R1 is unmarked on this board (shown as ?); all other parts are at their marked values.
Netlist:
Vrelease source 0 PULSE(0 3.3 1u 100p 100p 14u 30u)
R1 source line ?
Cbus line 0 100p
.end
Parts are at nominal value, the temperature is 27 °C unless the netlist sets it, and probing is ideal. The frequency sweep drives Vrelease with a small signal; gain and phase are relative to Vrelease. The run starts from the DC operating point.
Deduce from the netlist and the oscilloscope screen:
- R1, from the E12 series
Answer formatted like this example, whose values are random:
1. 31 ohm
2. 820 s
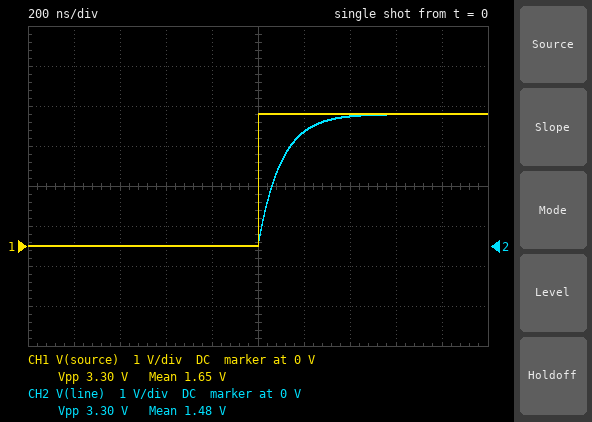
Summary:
1. 1 kΩ
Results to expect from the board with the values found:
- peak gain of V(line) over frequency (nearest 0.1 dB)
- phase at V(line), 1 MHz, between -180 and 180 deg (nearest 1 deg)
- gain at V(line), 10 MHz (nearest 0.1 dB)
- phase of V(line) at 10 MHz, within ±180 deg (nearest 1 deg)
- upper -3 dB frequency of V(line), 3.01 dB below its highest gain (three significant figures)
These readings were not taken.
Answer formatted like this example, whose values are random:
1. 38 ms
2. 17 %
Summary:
1. 0 dB
2. -32 deg
3. -16.1 dB
4. -81 deg
5. 1.59 MHz
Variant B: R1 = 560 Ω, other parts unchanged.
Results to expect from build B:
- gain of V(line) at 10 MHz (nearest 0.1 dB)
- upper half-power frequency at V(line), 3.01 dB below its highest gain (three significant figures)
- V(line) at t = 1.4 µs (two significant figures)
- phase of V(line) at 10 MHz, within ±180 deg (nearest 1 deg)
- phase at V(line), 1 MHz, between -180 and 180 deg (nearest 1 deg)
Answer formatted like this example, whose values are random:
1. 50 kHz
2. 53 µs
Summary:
1. -11.3 dB
2. 2.84 MHz
3. 3.3 V
4. -74 deg
5. -19 deg
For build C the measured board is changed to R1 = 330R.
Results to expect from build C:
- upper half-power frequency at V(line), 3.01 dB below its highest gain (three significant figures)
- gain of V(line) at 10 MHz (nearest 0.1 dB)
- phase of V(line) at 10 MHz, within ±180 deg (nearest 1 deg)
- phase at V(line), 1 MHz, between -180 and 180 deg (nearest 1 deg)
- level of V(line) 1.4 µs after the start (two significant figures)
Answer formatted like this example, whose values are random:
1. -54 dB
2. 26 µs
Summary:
1. 4.82 MHz
2. -7.2 dB
3. -64 deg
4. -12 deg
5. 3.3 V
